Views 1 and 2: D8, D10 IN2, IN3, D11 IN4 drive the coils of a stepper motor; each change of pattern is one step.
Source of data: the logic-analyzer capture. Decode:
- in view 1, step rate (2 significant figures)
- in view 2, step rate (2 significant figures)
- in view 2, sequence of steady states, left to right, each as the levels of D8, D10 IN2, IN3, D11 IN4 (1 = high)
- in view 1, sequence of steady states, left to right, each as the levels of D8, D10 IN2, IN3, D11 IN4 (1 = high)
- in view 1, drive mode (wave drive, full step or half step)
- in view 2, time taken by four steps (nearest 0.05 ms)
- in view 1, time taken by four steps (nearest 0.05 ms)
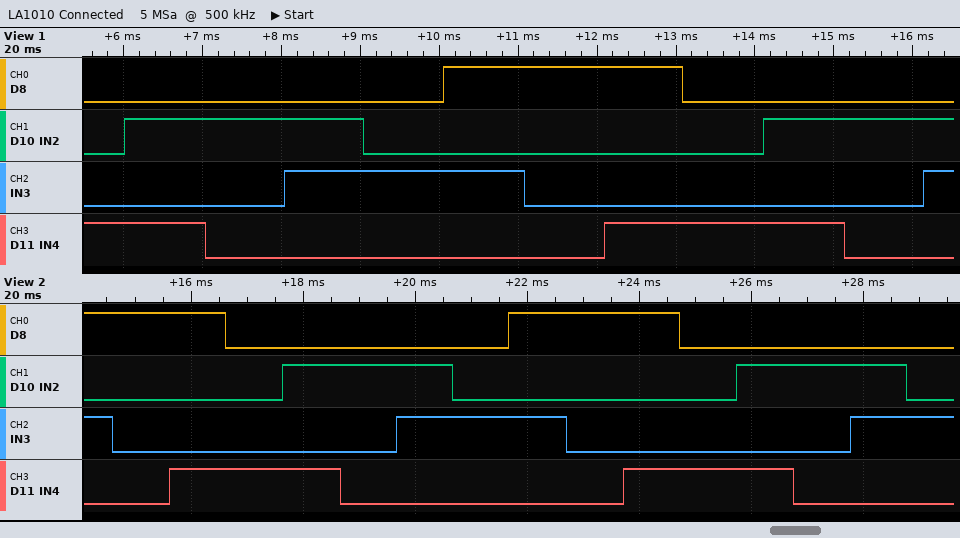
990 steps/s
990 steps/s
1010 1000 1001 0001 0101 0100 0110 0010 1010 1000 1001 0001 0101 0100 0110 0010
0001 0101 0100 0110 0010 1010 1000 1001 0001 0101 0100 0110
half step
4.05 ms
4.05 ms
